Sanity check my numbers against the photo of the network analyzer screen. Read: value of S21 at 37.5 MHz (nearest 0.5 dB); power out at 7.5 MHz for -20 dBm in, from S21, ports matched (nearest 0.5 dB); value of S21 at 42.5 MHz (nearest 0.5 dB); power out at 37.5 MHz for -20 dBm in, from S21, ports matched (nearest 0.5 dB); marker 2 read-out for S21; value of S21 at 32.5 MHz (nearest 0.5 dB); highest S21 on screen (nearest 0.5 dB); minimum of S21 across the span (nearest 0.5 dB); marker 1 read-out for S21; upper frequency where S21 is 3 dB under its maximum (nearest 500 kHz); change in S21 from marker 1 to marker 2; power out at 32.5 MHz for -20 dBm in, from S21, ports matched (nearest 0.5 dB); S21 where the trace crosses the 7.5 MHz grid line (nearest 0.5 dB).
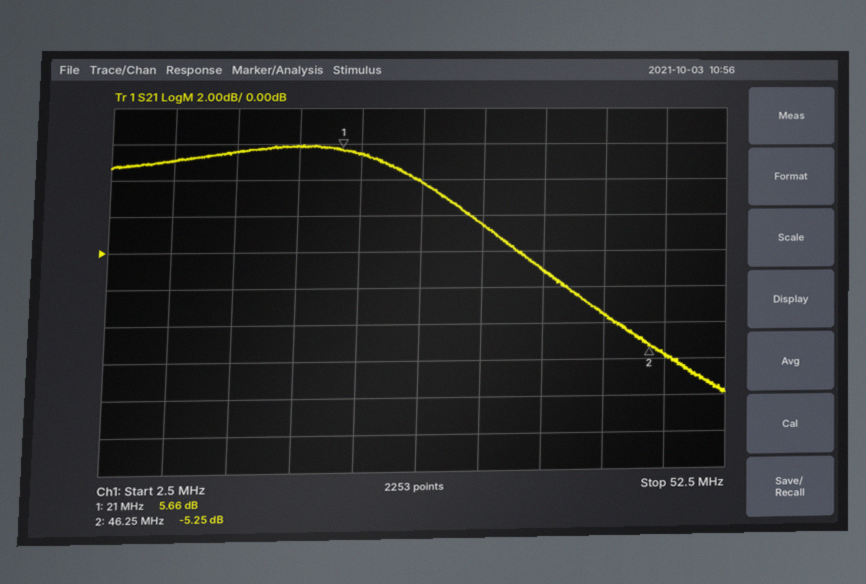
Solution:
-1.0 dB
-15.0 dBm
-3.5 dB
-21.0 dBm
-5.25 dB
1.5 dB
6.0 dB
-8.0 dB
5.66 dB
29.5 MHz
-10.91 dB
-18.5 dBm
5.0 dB
